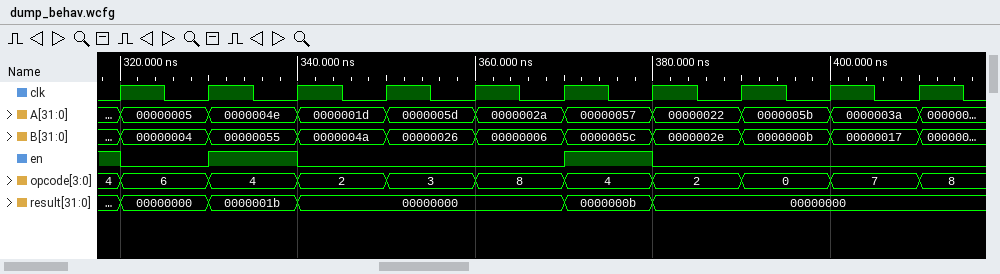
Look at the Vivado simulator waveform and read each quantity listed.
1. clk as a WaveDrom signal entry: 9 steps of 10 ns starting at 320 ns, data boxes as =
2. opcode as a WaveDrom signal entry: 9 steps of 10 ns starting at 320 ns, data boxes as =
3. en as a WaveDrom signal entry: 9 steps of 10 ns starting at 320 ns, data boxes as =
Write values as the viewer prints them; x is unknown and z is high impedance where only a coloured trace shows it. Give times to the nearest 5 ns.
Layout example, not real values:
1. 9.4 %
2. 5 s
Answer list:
1. {name: 'clk', wave: 'p........'}
2. {name: 'opcode', wave: '=========', data: '6 4 2 3 8 4 2 0 7'}
3. {name: 'en', wave: '010..10..'}
